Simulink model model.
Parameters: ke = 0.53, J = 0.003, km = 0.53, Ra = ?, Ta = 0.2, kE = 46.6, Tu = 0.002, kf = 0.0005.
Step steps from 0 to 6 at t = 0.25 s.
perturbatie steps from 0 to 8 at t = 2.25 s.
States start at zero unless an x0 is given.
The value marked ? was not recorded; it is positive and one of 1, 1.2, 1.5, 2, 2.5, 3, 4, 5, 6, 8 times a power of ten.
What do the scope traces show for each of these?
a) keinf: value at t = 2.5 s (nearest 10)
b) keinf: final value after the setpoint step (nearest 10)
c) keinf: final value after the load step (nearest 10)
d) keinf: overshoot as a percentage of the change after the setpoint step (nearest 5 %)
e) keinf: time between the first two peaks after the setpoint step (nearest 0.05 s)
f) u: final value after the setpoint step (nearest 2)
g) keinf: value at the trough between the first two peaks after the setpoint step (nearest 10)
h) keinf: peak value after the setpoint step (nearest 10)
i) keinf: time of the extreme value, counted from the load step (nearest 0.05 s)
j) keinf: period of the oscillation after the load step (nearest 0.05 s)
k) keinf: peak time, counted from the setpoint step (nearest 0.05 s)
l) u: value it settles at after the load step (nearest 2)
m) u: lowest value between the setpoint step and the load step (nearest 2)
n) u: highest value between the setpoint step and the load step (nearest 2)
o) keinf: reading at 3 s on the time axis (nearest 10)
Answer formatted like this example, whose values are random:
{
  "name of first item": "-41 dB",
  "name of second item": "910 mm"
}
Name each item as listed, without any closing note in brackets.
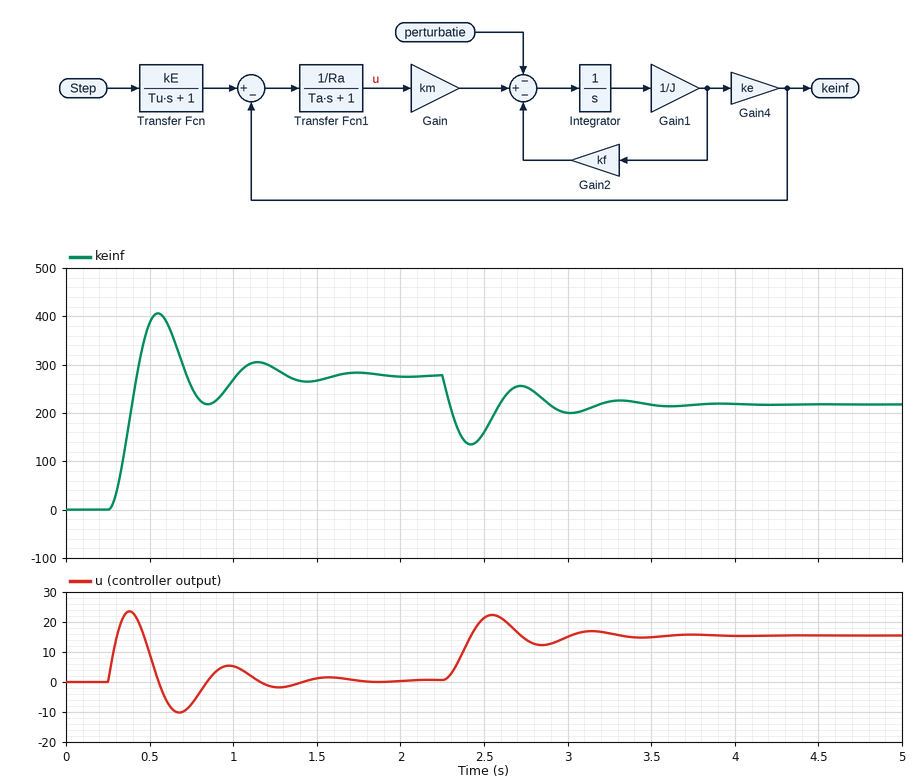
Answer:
{
  "keinf: value at t = 2.5 s": "160",
  "keinf: final value after the setpoint step": "280",
  "keinf: final value after the load step": "220",
  "keinf: overshoot as a percentage of the change after the setpoint step": "45 %",
  "keinf: time between the first two peaks after the setpoint step": "0.60 s",
  "u: final value after the setpoint step": "0",
  "keinf: value at the trough between the first two peaks after the setpoint step": "220",
  "keinf: peak value after the setpoint step": "410",
  "keinf: time of the extreme value, counted from the load step": "0.15 s",
  "keinf: period of the oscillation after the load step": "0.60 s",
  "keinf: peak time, counted from the setpoint step": "0.30 s",
  "u: value it settles at after the load step": "16",
  "u: lowest value between the setpoint step and the load step": "-10",
  "u: highest value between the setpoint step and the load step": "24",
  "keinf: reading at 3 s on the time axis": "200"
}
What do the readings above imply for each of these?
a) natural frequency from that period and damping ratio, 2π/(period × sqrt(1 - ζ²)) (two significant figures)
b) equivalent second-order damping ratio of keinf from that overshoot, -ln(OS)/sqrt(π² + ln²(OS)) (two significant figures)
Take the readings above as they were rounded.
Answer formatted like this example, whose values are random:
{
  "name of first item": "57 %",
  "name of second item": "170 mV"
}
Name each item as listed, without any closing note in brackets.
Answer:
{
  "natural frequency from that period and damping ratio, 2π/(period × sqrt(1 - ζ²))": "11 rad/s",
  "equivalent second-order damping ratio of keinf from that overshoot, -ln(OS)/sqrt(π² + ln²(OS))": "0.25"
}
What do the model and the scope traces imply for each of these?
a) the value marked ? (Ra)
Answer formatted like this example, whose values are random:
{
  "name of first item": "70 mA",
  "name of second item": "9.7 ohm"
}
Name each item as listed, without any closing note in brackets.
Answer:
{
  "the value marked ?": "4"
}
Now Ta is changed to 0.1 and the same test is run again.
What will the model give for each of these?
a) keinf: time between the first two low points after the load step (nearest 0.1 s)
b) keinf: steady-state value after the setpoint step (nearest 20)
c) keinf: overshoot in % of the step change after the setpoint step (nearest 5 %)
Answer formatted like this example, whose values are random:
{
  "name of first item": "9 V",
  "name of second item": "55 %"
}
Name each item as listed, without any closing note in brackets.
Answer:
{
  "keinf: time between the first two low points after the load step": "0.4 s",
  "keinf: steady-state value after the setpoint step": "280",
  "keinf: overshoot in % of the step change after the setpoint step": "35 %"
}
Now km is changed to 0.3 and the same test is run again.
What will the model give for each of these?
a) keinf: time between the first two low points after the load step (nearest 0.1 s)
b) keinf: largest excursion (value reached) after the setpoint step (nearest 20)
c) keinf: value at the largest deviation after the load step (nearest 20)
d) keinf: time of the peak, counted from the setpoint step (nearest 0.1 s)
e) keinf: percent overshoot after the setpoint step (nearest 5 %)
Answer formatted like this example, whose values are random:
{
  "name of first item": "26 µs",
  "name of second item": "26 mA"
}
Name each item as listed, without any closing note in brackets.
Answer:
{
  "keinf: time between the first two low points after the load step": "0.8 s",
  "keinf: largest excursion (value reached) after the setpoint step": "380",
  "keinf: value at the largest deviation after the load step": "80",
  "keinf: time of the peak, counted from the setpoint step": "0.4 s",
  "keinf: percent overshoot after the setpoint step": "35 %"
}
